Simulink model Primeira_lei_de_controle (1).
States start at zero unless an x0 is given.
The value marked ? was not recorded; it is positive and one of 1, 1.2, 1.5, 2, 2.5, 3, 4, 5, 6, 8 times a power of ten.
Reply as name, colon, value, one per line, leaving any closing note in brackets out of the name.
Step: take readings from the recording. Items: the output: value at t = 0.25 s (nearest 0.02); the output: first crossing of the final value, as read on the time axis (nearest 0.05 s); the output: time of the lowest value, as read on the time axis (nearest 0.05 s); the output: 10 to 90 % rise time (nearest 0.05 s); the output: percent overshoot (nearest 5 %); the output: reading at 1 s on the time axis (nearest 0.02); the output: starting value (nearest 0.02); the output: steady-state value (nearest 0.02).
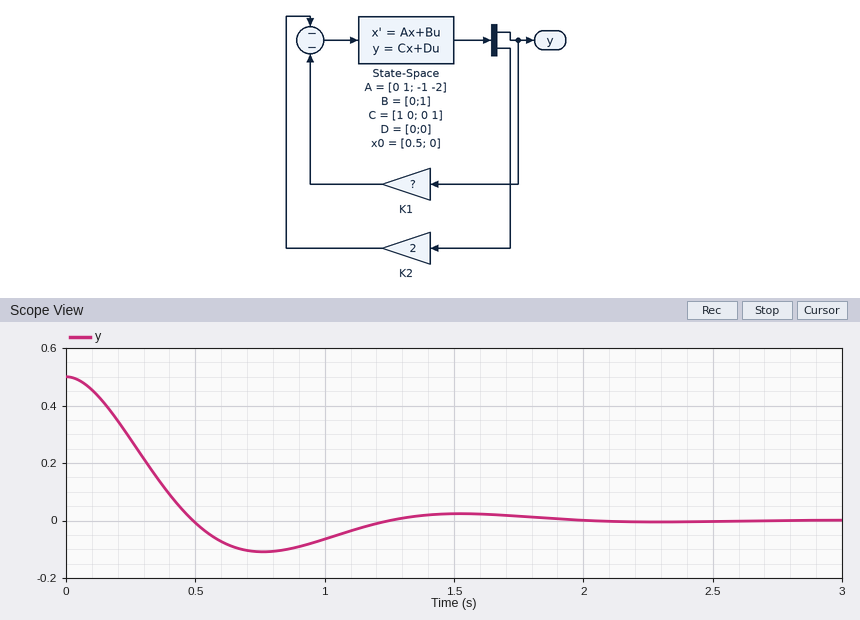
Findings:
the output: value at t = 0.25 s: 0.28
the output: first crossing of the final value, as read on the time axis: 0.50 s
the output: time of the lowest value, as read on the time axis: 0.75 s
the output: 10 to 90 % rise time: 0.35 s
the output: percent overshoot: 20 %
the output: reading at 1 s on the time axis: -0.06
the output: starting value: 0.50
the output: steady-state value: 0.00
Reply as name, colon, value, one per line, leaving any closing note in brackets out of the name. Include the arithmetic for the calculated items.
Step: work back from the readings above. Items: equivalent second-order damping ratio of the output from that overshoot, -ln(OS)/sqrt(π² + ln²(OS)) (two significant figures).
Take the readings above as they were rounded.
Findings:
equivalent second-order damping ratio of the output from that overshoot, -ln(OS)/sqrt(π² + ln²(OS)): ln(0.2) = -1.609; 1.609 / sqrt(9.870 + 2.590) = 0.46
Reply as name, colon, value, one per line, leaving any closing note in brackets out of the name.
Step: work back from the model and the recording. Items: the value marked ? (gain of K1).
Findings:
the value marked ?: 20
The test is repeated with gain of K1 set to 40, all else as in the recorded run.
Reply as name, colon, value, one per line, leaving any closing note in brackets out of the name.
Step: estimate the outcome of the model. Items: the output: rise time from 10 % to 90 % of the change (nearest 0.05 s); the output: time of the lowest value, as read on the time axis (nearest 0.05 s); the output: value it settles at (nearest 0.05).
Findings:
the output: rise time from 10 % to 90 % of the change: 0.20 s
the output: time of the lowest value, as read on the time axis: 0.50 s
the output: value it settles at: 0.00
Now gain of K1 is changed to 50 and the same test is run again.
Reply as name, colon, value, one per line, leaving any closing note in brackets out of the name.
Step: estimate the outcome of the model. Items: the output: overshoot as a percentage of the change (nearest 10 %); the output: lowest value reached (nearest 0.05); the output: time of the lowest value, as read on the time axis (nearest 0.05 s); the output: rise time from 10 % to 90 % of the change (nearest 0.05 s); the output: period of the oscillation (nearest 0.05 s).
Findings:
the output: overshoot as a percentage of the change: 40 %
the output: lowest value reached: -0.20
the output: time of the lowest value, as read on the time axis: 0.45 s
the output: rise time from 10 % to 90 % of the change: 0.20 s
the output: period of the oscillation: 0.90 s
